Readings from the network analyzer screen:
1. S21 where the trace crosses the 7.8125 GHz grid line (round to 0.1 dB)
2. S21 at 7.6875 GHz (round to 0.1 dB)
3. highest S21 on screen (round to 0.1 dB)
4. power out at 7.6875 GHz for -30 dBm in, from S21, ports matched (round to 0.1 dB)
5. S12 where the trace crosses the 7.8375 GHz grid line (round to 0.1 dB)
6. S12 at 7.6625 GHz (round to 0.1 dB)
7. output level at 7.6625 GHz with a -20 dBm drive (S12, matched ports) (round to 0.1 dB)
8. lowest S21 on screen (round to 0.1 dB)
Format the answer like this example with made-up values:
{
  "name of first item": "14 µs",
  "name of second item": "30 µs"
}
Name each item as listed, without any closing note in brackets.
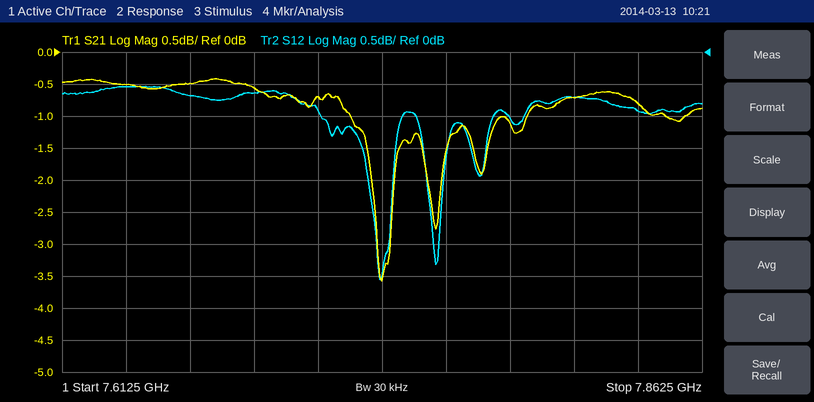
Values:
{
  "S21 where the trace crosses the 7.8125 GHz grid line": "-0.7 dB",
  "S21 at 7.6875 GHz": "-0.6 dB",
  "highest S21 on screen": "-0.4 dB",
  "power out at 7.6875 GHz for -30 dBm in, from S21, ports matched": "-30.6 dBm",
  "S12 where the trace crosses the 7.8375 GHz grid line": "-0.9 dB",
  "S12 at 7.6625 GHz": "-0.7 dB",
  "output level at 7.6625 GHz with a -20 dBm drive (S12, matched ports)": "-20.7 dBm",
  "lowest S21 on screen": "-3.6 dB"
}
